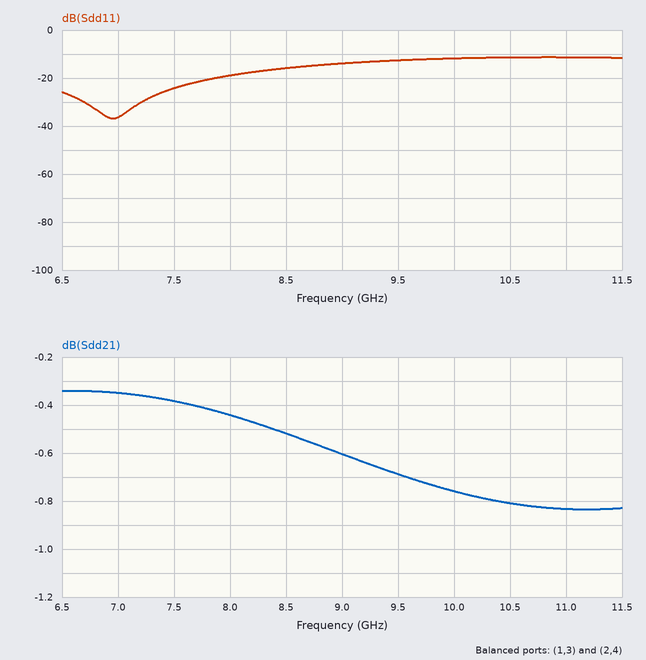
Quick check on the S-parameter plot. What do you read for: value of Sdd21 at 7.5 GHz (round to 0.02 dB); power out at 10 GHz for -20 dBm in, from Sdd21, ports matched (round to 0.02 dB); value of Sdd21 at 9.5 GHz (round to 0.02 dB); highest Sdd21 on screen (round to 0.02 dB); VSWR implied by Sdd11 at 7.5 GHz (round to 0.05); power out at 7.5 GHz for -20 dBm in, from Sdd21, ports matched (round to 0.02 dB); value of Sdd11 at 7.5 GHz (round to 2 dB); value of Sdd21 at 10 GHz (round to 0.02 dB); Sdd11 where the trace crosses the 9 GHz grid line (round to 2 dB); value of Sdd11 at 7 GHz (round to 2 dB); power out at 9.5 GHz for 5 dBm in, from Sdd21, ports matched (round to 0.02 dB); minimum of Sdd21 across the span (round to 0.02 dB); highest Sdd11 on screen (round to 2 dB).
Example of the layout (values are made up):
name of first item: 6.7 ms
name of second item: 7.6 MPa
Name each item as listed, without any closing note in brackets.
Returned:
value of Sdd21 at 7.5 GHz: -0.38 dB
power out at 10 GHz for -20 dBm in, from Sdd21, ports matched: -20.76 dBm
value of Sdd21 at 9.5 GHz: -0.68 dB
highest Sdd21 on screen: -0.34 dB
VSWR implied by Sdd11 at 7.5 GHz: 1.15
power out at 7.5 GHz for -20 dBm in, from Sdd21, ports matched: -20.38 dBm
value of Sdd11 at 7.5 GHz: -24 dB
value of Sdd21 at 10 GHz: -0.76 dB
Sdd11 where the trace crosses the 9 GHz grid line: -14 dB
value of Sdd11 at 7 GHz: -36 dB
power out at 9.5 GHz for 5 dBm in, from Sdd21, ports matched: 4.32 dBm
minimum of Sdd21 across the span: -0.84 dB
highest Sdd11 on screen: -12 dB
